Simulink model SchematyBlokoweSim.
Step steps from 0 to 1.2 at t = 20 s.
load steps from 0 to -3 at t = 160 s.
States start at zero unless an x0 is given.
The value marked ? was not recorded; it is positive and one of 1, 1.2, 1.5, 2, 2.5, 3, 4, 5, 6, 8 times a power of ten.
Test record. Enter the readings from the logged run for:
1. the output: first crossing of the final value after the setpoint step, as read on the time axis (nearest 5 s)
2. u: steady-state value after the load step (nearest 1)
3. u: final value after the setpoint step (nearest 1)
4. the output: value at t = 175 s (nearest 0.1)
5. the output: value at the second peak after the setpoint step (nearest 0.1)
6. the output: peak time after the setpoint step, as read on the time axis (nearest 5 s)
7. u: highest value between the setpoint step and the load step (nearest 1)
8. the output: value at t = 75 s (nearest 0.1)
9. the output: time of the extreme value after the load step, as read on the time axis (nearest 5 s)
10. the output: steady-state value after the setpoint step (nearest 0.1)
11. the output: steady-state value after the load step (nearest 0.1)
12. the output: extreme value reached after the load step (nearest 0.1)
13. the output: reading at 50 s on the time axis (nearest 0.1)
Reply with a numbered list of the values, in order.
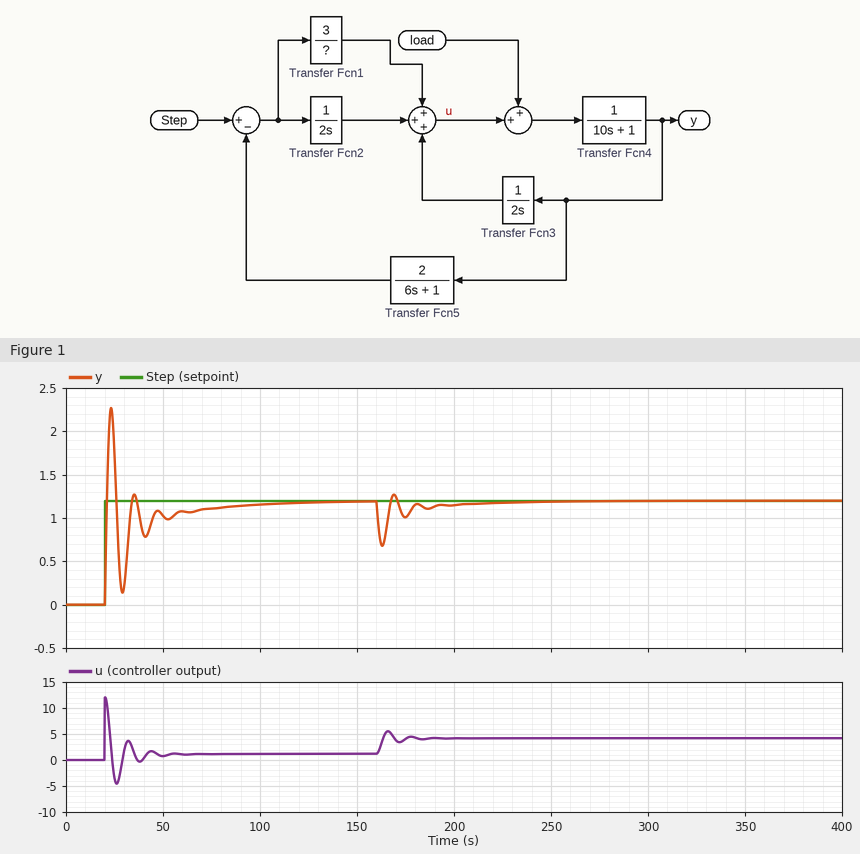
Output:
1. 20 s
2. 4
3. 1
4. 1.0
5. 1.3
6. 25 s
7. 12
8. 1.1
9. 165 s
10. 1.2
11. 1.2
12. 0.7
13. 1.0
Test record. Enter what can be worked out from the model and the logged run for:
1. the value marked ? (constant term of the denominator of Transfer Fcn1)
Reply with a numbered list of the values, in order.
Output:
1. 0.3
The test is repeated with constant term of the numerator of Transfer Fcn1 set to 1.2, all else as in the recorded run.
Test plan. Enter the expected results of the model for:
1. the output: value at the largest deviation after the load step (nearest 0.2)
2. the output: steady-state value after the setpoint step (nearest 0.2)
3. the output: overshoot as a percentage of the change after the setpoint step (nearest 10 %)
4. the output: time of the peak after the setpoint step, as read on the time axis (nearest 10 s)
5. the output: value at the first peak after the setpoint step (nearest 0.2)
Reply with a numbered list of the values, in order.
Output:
1. 0.4
2. 1.2
3. 70 %
4. 30 s
5. 2.0
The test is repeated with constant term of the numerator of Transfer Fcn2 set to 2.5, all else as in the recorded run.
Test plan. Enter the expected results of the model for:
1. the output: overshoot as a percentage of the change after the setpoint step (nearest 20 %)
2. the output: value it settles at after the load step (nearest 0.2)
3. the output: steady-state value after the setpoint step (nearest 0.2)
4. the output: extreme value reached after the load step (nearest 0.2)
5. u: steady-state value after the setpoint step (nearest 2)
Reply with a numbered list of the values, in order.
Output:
1. 240 %
2. 0.8
3. 0.8
4. 0.2
5. 0
